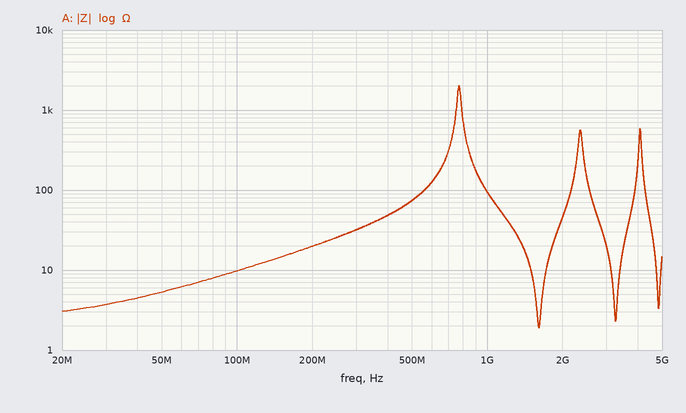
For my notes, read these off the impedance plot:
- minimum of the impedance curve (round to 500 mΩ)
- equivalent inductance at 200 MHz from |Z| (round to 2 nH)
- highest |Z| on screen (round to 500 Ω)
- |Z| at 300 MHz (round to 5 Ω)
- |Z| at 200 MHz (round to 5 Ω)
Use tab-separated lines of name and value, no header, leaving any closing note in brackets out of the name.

minimum of the impedance curve	2.0 Ω
equivalent inductance at 200 MHz from |Z|	16 nH
highest |Z| on screen	2.0 kΩ
|Z| at 300 MHz	30 Ω
|Z| at 200 MHz	20 Ω
